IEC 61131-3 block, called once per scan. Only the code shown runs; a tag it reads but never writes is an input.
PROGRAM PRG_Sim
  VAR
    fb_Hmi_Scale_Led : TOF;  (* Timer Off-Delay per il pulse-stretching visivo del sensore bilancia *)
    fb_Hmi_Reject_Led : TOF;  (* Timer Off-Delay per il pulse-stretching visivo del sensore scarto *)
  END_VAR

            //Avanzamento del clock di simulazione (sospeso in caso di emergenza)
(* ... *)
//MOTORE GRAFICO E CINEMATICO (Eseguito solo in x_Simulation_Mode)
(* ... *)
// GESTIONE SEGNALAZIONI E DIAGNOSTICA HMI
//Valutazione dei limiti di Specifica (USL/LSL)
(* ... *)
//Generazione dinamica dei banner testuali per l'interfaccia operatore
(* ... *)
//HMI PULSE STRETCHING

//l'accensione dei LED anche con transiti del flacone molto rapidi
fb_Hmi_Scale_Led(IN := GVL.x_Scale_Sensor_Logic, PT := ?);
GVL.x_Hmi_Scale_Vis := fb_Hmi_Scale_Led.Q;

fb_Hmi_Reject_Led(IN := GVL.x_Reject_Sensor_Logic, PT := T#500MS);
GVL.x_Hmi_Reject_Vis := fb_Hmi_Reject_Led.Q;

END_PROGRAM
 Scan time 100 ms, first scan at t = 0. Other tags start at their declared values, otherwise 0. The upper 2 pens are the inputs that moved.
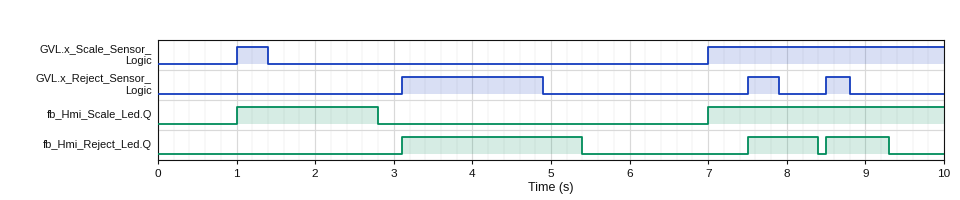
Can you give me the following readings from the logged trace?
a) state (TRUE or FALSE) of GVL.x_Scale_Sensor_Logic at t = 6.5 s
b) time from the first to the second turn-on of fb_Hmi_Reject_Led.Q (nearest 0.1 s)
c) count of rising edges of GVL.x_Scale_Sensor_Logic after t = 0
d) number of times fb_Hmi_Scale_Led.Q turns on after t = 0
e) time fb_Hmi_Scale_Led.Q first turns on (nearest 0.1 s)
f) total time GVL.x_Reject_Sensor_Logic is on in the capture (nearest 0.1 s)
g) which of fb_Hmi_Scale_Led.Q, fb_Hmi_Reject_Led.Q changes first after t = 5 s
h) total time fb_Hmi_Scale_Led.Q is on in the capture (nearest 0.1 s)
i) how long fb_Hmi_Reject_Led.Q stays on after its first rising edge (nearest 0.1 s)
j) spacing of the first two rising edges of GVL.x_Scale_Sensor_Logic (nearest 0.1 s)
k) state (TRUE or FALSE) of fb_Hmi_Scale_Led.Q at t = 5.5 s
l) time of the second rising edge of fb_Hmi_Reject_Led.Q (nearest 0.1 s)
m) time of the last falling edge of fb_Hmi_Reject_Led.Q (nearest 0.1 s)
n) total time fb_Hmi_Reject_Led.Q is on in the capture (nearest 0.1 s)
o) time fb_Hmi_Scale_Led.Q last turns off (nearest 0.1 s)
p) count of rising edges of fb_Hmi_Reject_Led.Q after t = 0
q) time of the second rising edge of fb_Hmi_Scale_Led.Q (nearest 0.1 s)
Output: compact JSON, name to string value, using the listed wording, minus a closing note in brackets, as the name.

{"state (TRUE or FALSE) of GVL.x_Scale_Sensor_Logic at t = 6.5 s": "FALSE", "time from the first to the second turn-on of fb_Hmi_Reject_Led.Q": "4.4 s", "count of rising edges of GVL.x_Scale_Sensor_Logic after t = 0": "2", "number of times fb_Hmi_Scale_Led.Q turns on after t = 0": "2", "time fb_Hmi_Scale_Led.Q first turns on": "1.0 s", "total time GVL.x_Reject_Sensor_Logic is on in the capture": "2.5 s", "which of fb_Hmi_Scale_Led.Q, fb_Hmi_Reject_Led.Q changes first after t = 5 s": "fb_Hmi_Reject_Led.Q", "total time fb_Hmi_Scale_Led.Q is on in the capture": "4.8 s", "how long fb_Hmi_Reject_Led.Q stays on after its first rising edge": "2.3 s", "spacing of the first two rising edges of GVL.x_Scale_Sensor_Logic": "6.0 s", "state (TRUE or FALSE) of fb_Hmi_Scale_Led.Q at t = 5.5 s": "FALSE", "time of the second rising edge of fb_Hmi_Reject_Led.Q": "7.5 s", "time of the last falling edge of fb_Hmi_Reject_Led.Q": "9.3 s", "total time fb_Hmi_Reject_Led.Q is on in the capture": "4.0 s", "time fb_Hmi_Scale_Led.Q last turns off": "2.8 s", "count of rising edges of fb_Hmi_Reject_Led.Q after t = 0": "3", "time of the second rising edge of fb_Hmi_Scale_Led.Q": "7.0 s"}
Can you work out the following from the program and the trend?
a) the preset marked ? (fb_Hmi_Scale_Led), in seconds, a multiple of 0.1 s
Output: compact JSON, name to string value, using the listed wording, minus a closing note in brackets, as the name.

{"the preset marked ? (fb_Hmi_Scale_Led), in seconds, a multiple of 0.1 s": "1.4 s"}
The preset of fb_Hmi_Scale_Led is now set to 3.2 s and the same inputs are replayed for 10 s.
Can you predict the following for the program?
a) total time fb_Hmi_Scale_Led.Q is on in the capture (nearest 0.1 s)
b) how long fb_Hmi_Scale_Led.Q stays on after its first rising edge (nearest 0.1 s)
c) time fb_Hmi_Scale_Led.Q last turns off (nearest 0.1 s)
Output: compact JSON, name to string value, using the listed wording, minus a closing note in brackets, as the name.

{"total time fb_Hmi_Scale_Led.Q is on in the capture": "6.6 s", "how long fb_Hmi_Scale_Led.Q stays on after its first rising edge": "3.6 s", "time fb_Hmi_Scale_Led.Q last turns off": "4.6 s"}
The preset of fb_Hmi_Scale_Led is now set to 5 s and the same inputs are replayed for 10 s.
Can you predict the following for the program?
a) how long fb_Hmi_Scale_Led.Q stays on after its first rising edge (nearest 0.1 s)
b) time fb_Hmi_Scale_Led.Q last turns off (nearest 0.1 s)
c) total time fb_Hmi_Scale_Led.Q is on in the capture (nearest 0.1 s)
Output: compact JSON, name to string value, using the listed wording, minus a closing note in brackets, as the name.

{"how long fb_Hmi_Scale_Led.Q stays on after its first rising edge": "5.4 s", "time fb_Hmi_Scale_Led.Q last turns off": "6.4 s", "total time fb_Hmi_Scale_Led.Q is on in the capture": "8.4 s"}
